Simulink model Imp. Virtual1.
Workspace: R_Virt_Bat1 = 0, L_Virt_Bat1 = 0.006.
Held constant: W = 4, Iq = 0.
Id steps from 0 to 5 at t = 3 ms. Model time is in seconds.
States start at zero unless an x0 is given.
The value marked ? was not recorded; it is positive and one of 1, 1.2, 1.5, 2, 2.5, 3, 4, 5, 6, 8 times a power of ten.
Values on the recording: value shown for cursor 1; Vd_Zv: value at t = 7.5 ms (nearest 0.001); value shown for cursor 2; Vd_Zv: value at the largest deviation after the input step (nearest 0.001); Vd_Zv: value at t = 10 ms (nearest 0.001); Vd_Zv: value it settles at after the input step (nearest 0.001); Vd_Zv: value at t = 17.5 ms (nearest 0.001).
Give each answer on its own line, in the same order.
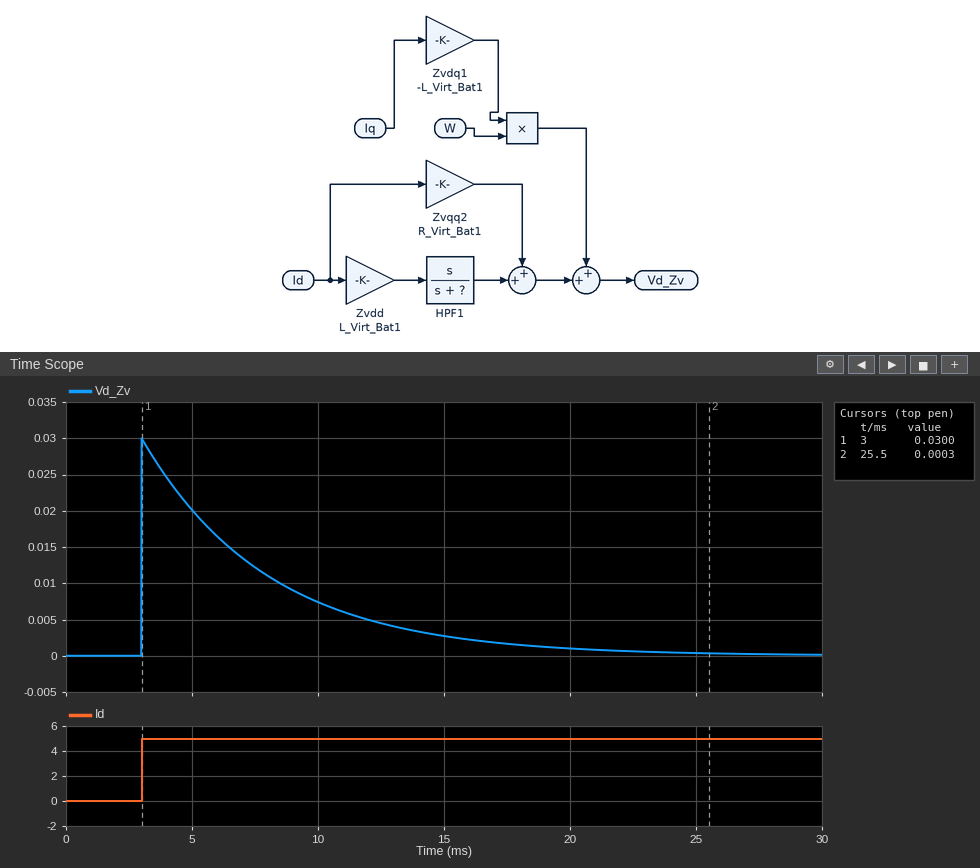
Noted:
0.0300
0.012
0.0003
0.030
0.007
0.000
0.002
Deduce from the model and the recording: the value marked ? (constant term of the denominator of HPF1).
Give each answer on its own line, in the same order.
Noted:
200
